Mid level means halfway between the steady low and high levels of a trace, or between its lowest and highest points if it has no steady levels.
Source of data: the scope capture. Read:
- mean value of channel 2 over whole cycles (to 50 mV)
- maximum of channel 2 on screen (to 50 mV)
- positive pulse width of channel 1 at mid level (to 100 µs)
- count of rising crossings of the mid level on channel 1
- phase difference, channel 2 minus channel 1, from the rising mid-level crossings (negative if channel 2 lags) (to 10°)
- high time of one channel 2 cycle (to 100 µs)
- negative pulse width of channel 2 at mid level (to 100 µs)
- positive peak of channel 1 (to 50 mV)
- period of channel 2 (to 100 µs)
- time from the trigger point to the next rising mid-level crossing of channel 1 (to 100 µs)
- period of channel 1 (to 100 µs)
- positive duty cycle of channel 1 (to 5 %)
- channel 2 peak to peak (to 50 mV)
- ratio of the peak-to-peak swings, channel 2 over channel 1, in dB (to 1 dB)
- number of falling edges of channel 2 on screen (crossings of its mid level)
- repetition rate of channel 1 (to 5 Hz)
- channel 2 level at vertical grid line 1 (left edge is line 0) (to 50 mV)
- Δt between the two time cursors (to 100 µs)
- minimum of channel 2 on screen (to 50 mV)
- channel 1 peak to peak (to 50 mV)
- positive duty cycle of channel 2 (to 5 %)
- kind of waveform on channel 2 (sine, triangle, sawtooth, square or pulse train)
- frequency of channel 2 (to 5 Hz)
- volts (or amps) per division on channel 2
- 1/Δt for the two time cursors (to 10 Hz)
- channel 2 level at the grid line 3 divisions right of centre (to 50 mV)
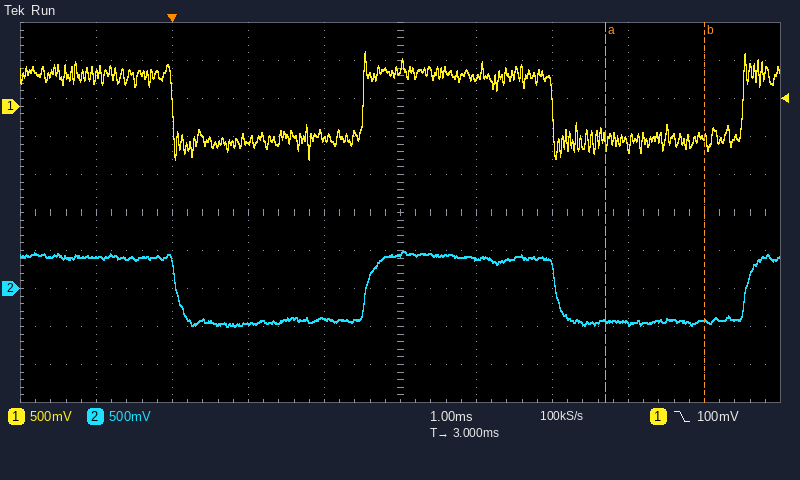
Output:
0 mV
500 mV
2.5 ms
2
0°
2.5 ms
2.5 ms
700 mV
5.0 ms
2.5 ms
5.0 ms
50 %
1.00 V
-3 dB
2
200 Hz
400 mV
1.3 ms
-500 mV
1.40 V
50 %
square
200 Hz
500 mV
770 Hz
-450 mV
